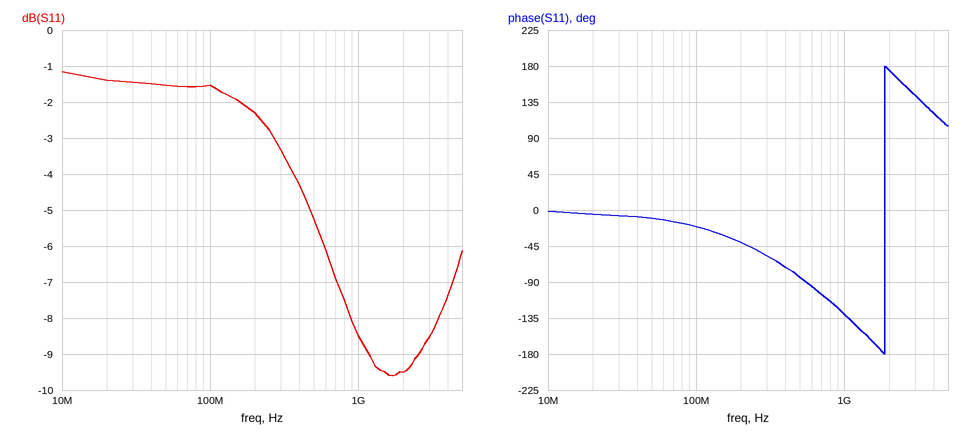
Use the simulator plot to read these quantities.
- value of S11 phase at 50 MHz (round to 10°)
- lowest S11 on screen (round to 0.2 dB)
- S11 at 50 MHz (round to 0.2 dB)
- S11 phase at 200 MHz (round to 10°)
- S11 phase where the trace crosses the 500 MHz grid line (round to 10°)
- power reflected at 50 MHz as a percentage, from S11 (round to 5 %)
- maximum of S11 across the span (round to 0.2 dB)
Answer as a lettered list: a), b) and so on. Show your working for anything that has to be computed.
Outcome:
a) -10°
b) -9.6 dB
c) -1.6 dB
d) -40°
e) -80°
f) 10^(-1.6/10) ≈ 69.2 %, so 70 % to the nearest 5 %
g) -1.2 dB
